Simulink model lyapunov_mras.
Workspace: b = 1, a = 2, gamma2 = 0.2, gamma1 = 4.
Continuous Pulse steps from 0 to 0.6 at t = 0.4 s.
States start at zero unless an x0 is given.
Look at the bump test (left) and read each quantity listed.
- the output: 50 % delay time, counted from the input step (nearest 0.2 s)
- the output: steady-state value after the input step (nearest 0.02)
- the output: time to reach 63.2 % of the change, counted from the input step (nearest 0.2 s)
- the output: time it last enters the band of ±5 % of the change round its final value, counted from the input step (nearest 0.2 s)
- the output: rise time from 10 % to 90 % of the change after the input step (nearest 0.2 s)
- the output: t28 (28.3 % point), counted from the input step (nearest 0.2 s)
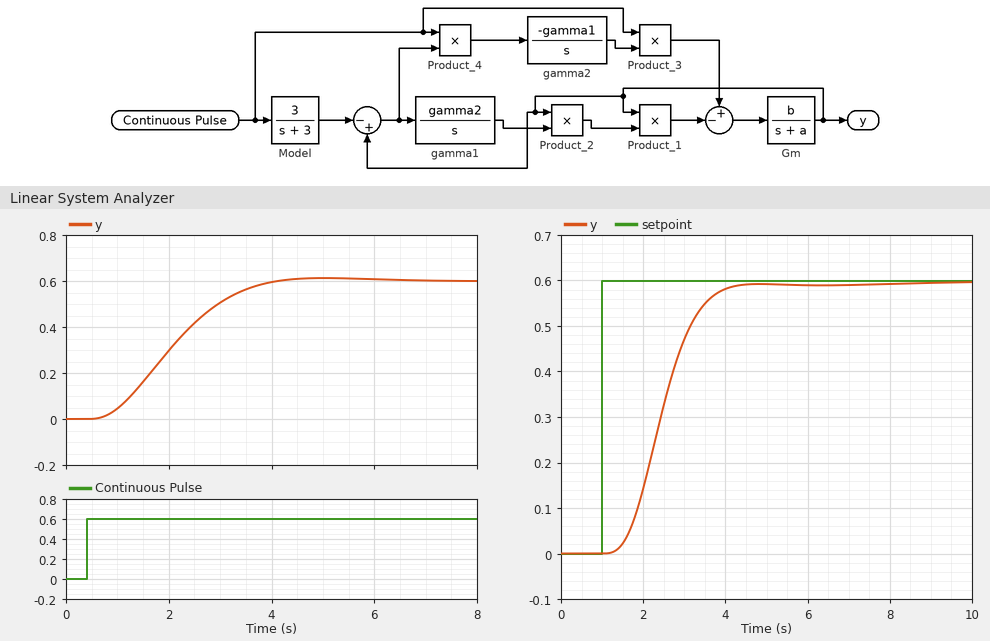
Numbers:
1.6 s
0.60
2.0 s
3.2 s
2.2 s
1.2 s
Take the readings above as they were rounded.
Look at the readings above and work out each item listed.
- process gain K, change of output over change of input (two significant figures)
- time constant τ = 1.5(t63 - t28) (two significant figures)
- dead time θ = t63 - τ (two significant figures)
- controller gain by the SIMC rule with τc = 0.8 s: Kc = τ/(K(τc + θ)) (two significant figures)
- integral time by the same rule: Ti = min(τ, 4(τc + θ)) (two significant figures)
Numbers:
1.0
1.2 s
0.80 s
0.75
1.2 s
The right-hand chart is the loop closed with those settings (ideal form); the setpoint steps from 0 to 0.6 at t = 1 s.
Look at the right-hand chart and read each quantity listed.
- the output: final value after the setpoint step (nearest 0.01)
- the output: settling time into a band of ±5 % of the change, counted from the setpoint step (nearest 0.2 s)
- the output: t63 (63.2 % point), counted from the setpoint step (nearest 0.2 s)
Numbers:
0.60
2.8 s
1.6 s
